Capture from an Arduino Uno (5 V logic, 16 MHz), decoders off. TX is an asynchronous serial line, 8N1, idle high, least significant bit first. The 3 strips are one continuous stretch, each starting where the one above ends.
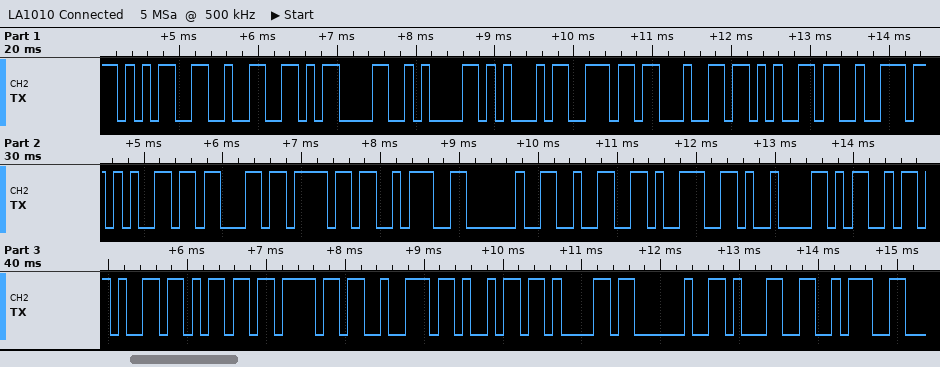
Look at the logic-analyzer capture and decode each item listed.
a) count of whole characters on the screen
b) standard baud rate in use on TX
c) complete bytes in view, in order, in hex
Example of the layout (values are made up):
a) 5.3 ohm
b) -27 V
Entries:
a) 27
b) 9600 baud
c) 0x35 0x32 0x0D 0x0A 0x45 0x6E 0x64 0x65 0x72 0x65 0x63 0x6F 0x3A 0x20 0x32 0x39 0x09 0x4D 0x65 0x6D 0x6F 0x72 0x69 0x61 0x20 0x31 0x3A
